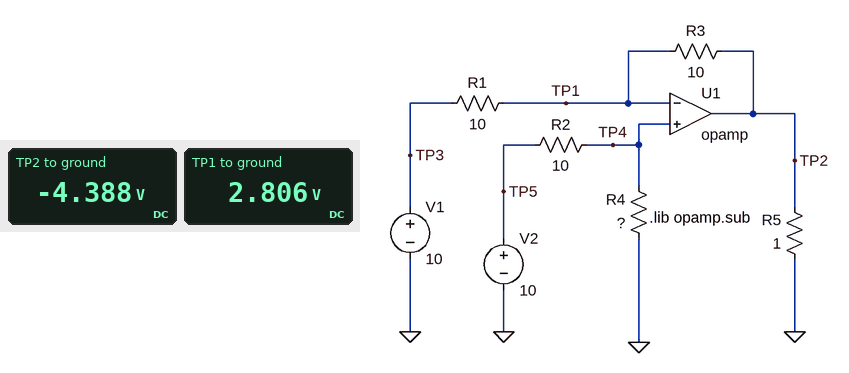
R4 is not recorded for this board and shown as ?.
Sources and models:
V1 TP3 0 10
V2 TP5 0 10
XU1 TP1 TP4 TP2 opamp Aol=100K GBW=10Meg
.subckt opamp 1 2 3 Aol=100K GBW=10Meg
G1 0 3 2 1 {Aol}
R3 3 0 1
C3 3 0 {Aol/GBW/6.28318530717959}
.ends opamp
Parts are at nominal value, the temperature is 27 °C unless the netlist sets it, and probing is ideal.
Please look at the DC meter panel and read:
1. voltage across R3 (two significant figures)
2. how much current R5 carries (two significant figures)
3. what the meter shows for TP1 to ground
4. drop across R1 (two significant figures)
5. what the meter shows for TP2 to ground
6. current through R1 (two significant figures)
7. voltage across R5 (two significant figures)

7.2 V
4.4 A
2.806 V
7.2 V
-4.388 V
720 mA
4.4 V
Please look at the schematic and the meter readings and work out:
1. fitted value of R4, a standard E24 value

3.9 Ω
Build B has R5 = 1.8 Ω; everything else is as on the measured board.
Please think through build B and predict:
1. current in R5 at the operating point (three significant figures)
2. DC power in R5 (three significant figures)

2.44 A
10.7 W
